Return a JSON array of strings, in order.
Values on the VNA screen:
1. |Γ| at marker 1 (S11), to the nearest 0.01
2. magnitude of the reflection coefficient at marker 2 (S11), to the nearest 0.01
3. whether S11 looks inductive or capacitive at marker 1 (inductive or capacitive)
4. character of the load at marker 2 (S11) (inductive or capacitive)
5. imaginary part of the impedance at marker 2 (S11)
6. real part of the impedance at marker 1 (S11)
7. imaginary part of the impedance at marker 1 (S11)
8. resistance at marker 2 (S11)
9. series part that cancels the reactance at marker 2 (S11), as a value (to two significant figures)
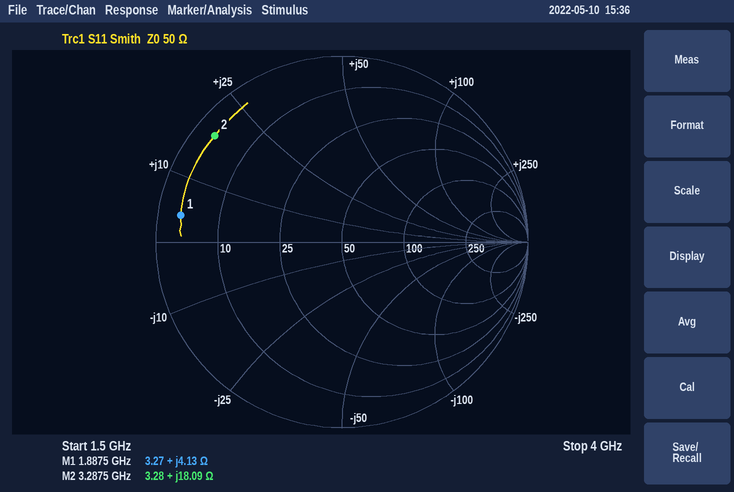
["0.88", "0.89", "inductive", "inductive", "+18.09 Ω", "3.27 Ω", "+4.13 Ω", "3.28 Ω", "2.7 pF"]
